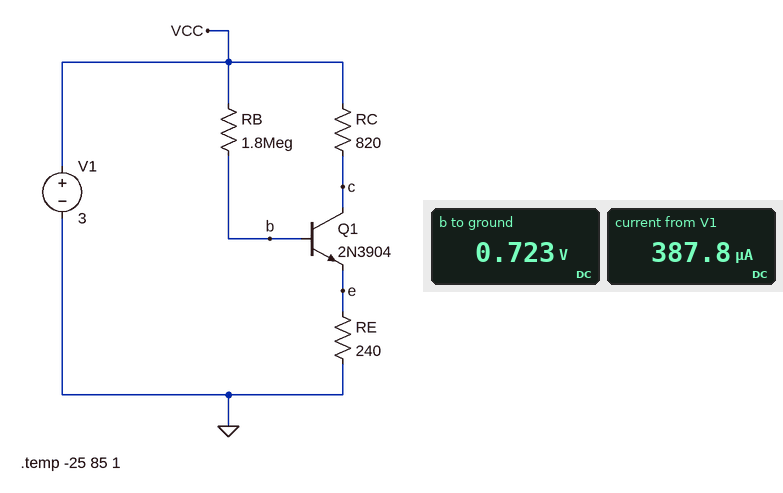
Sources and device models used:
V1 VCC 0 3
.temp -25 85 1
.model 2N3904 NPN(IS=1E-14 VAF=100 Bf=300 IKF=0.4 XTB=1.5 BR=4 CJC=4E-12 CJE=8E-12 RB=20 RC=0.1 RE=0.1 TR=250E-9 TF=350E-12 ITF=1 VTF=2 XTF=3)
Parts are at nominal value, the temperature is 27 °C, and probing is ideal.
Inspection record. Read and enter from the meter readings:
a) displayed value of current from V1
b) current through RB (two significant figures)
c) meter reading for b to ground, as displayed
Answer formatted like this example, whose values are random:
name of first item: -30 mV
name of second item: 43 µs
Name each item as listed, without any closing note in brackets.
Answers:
displayed value of current from V1: 387.8 µA
current through RB: 1.3 µA
meter reading for b to ground, as displayed: 0.723 V
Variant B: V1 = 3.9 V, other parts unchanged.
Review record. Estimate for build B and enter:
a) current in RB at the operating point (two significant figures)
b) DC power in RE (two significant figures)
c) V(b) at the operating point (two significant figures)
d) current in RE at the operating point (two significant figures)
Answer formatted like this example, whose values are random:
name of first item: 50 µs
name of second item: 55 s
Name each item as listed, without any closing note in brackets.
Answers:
current in RB at the operating point: 1.7 µA
DC power in RE: 69 µW
V(b) at the operating point: 770 mV
current in RE at the operating point: 540 µA
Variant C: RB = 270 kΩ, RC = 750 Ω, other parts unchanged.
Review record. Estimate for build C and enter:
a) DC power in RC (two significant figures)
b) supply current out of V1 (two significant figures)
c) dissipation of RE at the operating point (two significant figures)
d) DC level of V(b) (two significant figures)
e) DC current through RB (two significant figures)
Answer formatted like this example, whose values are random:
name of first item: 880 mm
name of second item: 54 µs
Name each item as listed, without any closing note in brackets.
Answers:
DC power in RC: 3.1 mW
supply current out of V1: 2.0 mA
dissipation of RE at the operating point: 1.0 mW
DC level of V(b): 1.2 V
DC current through RB: 6.8 µA
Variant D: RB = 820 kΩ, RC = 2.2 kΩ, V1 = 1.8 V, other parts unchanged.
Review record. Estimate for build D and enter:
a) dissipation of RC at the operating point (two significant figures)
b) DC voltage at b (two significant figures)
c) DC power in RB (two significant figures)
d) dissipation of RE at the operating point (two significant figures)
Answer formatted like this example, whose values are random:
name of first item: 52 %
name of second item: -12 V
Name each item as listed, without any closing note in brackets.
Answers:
dissipation of RC at the operating point: 340 µW
DC voltage at b: 730 mV
DC power in RB: 1.4 µW
dissipation of RE at the operating point: 37 µW
